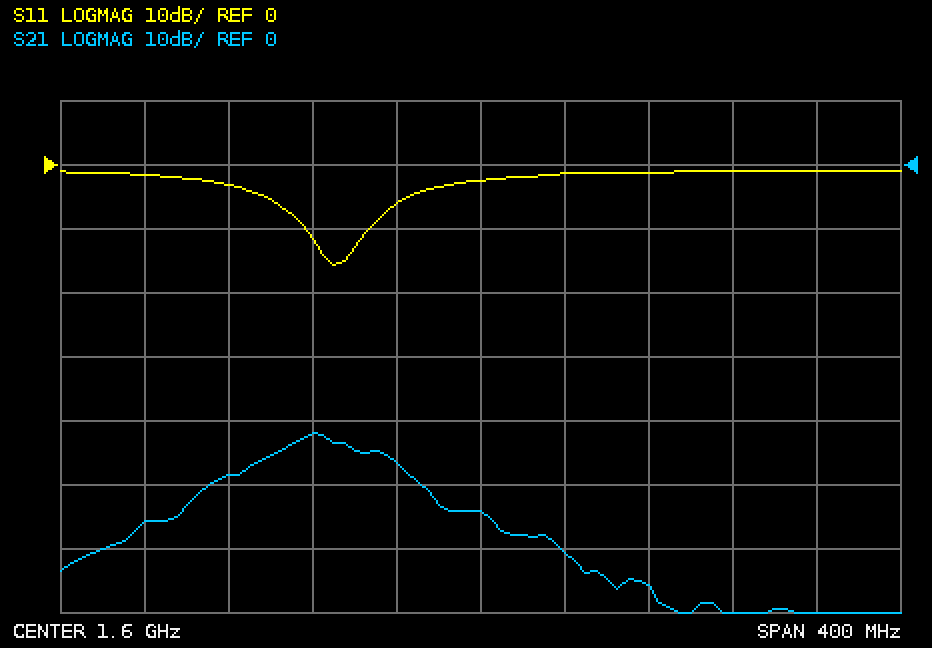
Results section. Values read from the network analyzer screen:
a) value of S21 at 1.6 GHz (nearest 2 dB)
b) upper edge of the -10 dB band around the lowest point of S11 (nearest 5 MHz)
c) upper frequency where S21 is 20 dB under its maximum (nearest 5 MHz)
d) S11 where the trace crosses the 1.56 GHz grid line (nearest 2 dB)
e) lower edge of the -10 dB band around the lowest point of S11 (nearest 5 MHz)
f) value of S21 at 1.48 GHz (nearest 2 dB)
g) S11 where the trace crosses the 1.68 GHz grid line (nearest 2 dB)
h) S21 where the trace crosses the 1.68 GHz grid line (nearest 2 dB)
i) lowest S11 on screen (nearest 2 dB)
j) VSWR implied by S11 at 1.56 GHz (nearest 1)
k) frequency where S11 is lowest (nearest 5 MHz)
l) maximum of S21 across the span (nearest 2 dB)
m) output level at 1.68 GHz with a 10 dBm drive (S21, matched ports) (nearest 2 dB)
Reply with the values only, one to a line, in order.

-54 dB
1.545 GHz
1.645 GHz
-6 dB
1.515 GHz
-48 dB
-2 dB
-66 dB
-16 dB
3
1.530 GHz
-42 dB
-56 dBm
